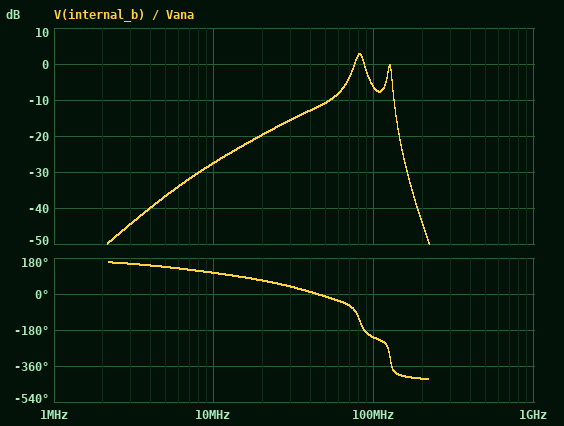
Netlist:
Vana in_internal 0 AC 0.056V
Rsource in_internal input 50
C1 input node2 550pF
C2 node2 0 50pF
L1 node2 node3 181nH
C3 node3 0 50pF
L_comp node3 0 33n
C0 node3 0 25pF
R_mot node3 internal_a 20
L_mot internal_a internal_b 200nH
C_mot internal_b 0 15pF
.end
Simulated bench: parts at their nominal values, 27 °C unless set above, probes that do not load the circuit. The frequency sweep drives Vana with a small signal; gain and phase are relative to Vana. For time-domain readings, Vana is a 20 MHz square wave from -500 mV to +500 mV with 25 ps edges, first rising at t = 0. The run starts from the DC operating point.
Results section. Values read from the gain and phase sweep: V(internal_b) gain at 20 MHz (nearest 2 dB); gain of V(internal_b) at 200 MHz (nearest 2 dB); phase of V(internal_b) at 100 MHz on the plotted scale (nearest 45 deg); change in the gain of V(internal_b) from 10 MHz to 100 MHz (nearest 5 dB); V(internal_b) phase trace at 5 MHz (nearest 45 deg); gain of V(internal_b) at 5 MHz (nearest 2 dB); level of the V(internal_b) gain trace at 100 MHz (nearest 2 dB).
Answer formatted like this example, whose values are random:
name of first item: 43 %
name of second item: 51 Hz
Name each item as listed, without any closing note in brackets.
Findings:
V(internal_b) gain at 20 MHz: -20 dB
gain of V(internal_b) at 200 MHz: -44 dB
phase of V(internal_b) at 100 MHz on the plotted scale: -225 deg
change in the gain of V(internal_b) from 10 MHz to 100 MHz: 20 dB
V(internal_b) phase trace at 5 MHz: 135 deg
gain of V(internal_b) at 5 MHz: -36 dB
level of the V(internal_b) gain trace at 100 MHz: -6 dB
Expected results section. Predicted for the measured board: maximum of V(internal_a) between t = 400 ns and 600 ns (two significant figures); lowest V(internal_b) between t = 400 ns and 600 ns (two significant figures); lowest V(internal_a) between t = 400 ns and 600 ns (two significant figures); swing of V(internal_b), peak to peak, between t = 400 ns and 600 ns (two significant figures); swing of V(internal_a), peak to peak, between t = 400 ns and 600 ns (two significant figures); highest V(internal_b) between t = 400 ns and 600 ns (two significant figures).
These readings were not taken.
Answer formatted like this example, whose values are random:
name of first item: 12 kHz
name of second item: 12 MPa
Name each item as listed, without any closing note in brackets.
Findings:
maximum of V(internal_a) between t = 400 ns and 600 ns: 130 mV
lowest V(internal_b) between t = 400 ns and 600 ns: -170 mV
lowest V(internal_a) between t = 400 ns and 600 ns: -130 mV
swing of V(internal_b), peak to peak, between t = 400 ns and 600 ns: 330 mV
swing of V(internal_a), peak to peak, between t = 400 ns and 600 ns: 250 mV
highest V(internal_b) between t = 400 ns and 600 ns: 170 mV
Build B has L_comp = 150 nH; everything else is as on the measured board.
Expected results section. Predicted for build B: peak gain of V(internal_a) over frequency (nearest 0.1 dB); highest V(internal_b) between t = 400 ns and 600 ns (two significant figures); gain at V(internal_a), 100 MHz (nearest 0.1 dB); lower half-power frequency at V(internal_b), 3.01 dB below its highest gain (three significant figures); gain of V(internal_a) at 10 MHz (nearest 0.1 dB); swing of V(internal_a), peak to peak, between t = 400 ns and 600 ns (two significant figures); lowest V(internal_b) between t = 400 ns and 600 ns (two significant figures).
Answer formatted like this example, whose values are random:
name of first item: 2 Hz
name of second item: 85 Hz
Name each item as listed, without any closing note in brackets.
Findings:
peak gain of V(internal_a) over frequency: 1.3 dB
highest V(internal_b) between t = 400 ns and 600 ns: 820 mV
gain at V(internal_a), 100 MHz: -16.7 dB
lower half-power frequency at V(internal_b), 3.01 dB below its highest gain: 51.4 MHz
gain of V(internal_a) at 10 MHz: -13.5 dB
swing of V(internal_a), peak to peak, between t = 400 ns and 600 ns: 1.0 V
lowest V(internal_b) between t = 400 ns and 600 ns: -820 mV
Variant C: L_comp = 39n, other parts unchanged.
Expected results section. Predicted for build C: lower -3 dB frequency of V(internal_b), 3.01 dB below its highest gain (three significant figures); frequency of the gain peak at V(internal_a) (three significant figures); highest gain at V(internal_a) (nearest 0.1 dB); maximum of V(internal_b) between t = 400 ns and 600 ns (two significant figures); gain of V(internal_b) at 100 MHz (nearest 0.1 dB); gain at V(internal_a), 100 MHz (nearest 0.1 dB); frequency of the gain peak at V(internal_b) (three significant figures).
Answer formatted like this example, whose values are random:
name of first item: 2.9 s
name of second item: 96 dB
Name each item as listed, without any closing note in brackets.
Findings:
lower -3 dB frequency of V(internal_b), 3.01 dB below its highest gain: 73.7 MHz
frequency of the gain peak at V(internal_a): 121 MHz
highest gain at V(internal_a): -2.9 dB
maximum of V(internal_b) between t = 400 ns and 600 ns: 200 mV
gain of V(internal_b) at 100 MHz: -5.4 dB
gain at V(internal_a), 100 MHz: -20.1 dB
frequency of the gain peak at V(internal_b): 79.2 MHz
